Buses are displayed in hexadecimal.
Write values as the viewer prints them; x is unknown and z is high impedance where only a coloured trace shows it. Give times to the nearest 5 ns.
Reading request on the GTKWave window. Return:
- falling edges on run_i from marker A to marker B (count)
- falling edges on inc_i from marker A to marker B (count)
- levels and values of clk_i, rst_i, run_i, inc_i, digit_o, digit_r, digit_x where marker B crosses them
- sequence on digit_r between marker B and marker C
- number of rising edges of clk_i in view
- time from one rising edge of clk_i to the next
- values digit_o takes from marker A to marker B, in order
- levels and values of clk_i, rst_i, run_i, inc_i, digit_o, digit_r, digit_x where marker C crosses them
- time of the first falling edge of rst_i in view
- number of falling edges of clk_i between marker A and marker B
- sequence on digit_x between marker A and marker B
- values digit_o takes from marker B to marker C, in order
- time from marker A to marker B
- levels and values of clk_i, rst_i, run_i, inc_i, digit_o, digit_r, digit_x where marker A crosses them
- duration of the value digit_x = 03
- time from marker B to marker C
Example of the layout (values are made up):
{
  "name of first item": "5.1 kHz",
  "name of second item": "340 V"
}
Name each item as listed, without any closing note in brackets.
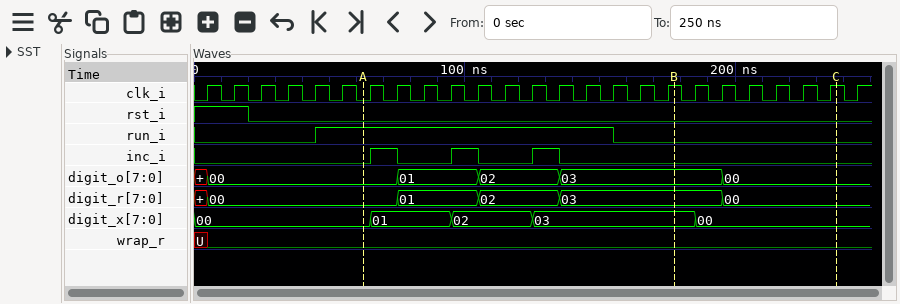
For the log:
{
  "falling edges on run_i from marker A to marker B": "1",
  "falling edges on inc_i from marker A to marker B": "3",
  "levels and values of clk_i, rst_i, run_i, inc_i, digit_o, digit_r, digit_x where marker B crosses them": "clk_i=1, rst_i=0, run_i=0, inc_i=0, digit_o=03, digit_r=03, digit_x=03",
  "sequence on digit_r between marker B and marker C": "03, 00",
  "number of rising edges of clk_i in view": "25",
  "time from one rising edge of clk_i to the next": "10 ns",
  "values digit_o takes from marker A to marker B, in order": "00, 01, 02, 03",
  "levels and values of clk_i, rst_i, run_i, inc_i, digit_o, digit_r, digit_x where marker C crosses them": "clk_i=1, rst_i=0, run_i=0, inc_i=0, digit_o=00, digit_r=00, digit_x=00",
  "time of the first falling edge of rst_i in view": "20 ns",
  "number of falling edges of clk_i between marker A and marker B": "11",
  "sequence on digit_x between marker A and marker B": "00, 01, 02, 03",
  "values digit_o takes from marker B to marker C, in order": "03, 00",
  "time from marker A to marker B": "115 ns",
  "levels and values of clk_i, rst_i, run_i, inc_i, digit_o, digit_r, digit_x where marker A crosses them": "clk_i=0, rst_i=0, run_i=1, inc_i=0, digit_o=00, digit_r=00, digit_x=00",
  "duration of the value digit_x = 03": "60 ns",
  "time from marker B to marker C": "60 ns"
}
